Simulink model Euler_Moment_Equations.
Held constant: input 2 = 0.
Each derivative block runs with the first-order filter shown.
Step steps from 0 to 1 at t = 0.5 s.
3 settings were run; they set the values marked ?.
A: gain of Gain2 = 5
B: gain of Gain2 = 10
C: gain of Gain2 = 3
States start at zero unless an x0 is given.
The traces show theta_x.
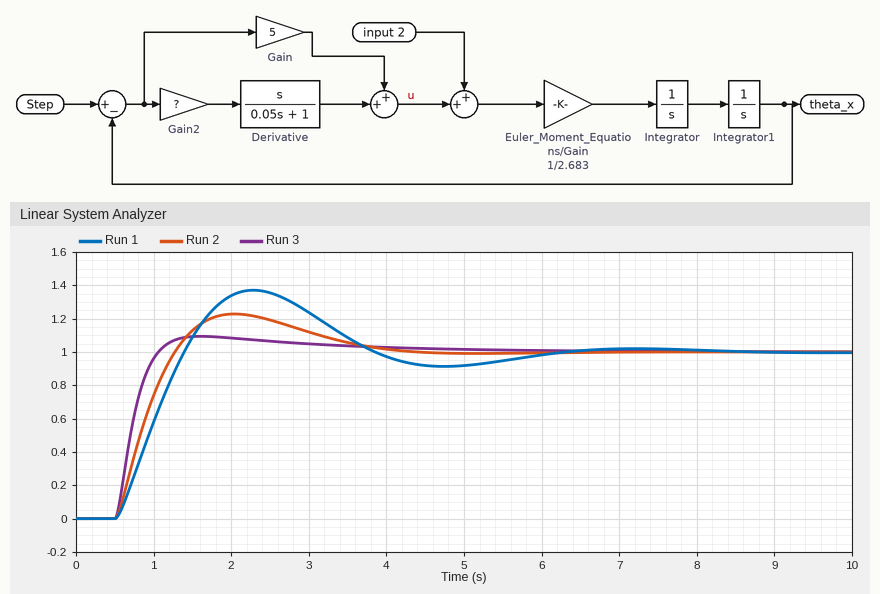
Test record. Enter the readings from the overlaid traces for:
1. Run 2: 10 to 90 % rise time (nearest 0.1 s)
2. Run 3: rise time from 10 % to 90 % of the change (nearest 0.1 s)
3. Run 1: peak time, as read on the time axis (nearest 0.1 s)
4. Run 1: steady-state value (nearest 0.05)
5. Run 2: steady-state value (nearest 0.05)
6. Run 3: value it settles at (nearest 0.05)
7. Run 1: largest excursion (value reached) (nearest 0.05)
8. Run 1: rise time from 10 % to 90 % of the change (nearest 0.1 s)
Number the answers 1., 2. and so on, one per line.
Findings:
1. 0.6 s
2. 0.4 s
3. 2.3 s
4. 1.00
5. 1.00
6. 1.00
7. 1.35
8. 0.7 s
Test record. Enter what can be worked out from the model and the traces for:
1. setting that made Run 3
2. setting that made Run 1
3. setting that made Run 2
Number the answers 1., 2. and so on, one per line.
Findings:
1. B
2. C
3. A
